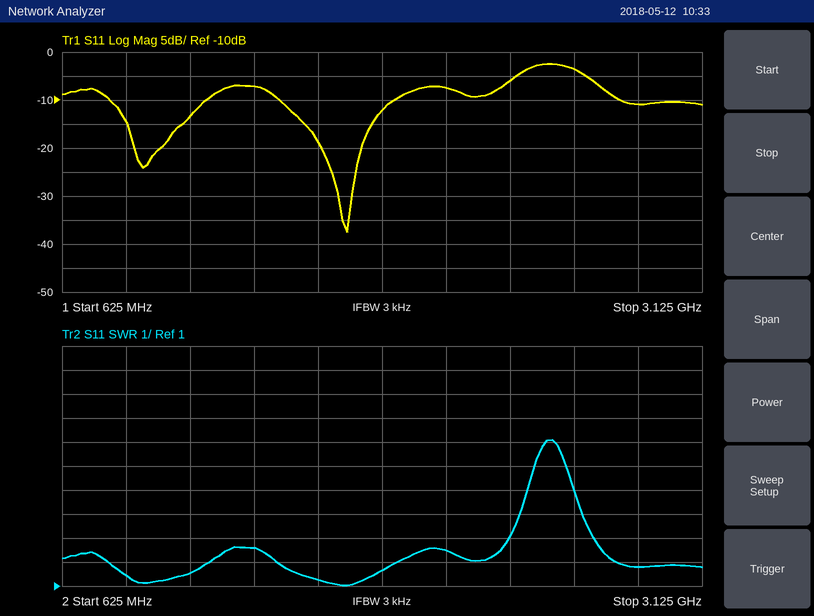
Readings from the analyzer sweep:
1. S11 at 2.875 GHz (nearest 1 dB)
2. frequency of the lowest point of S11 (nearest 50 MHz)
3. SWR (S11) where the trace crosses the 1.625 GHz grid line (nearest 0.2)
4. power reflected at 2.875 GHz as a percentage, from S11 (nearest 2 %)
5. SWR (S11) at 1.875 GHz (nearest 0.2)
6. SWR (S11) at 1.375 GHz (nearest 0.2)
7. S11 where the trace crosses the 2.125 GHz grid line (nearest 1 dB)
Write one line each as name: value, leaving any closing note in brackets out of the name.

S11 at 2.875 GHz: -11 dB
frequency of the lowest point of S11: 1.75 GHz
SWR (S11) where the trace crosses the 1.625 GHz grid line: 1.2
power reflected at 2.875 GHz as a percentage, from S11: 8 %
SWR (S11) at 1.875 GHz: 1.6
SWR (S11) at 1.375 GHz: 2.6
S11 where the trace crosses the 2.125 GHz grid line: -7 dB
